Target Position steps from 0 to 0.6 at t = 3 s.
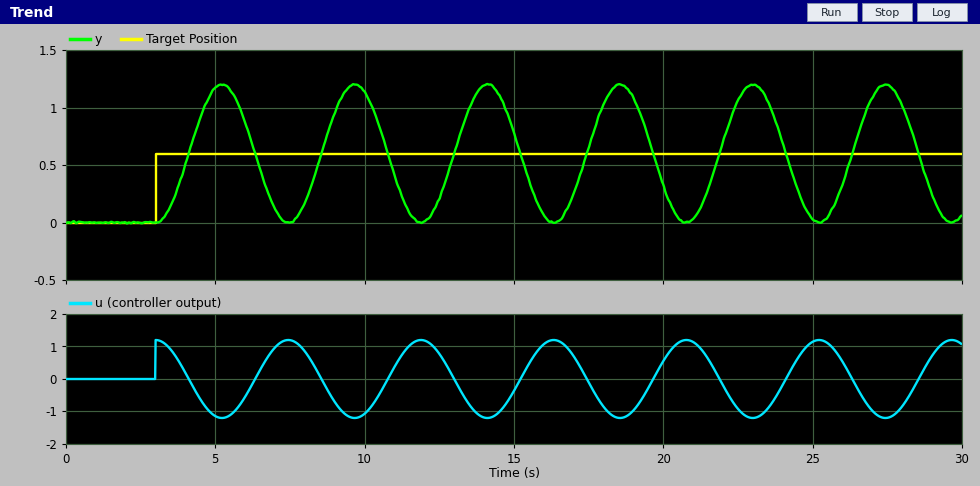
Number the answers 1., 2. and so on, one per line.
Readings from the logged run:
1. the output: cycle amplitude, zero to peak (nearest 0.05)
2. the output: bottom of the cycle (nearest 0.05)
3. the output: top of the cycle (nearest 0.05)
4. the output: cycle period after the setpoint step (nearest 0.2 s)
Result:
1. 0.60
2. 0.00
3. 1.20
4. 4.4 s
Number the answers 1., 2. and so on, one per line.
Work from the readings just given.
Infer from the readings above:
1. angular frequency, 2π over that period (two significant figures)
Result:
1. 1.4 rad/s
